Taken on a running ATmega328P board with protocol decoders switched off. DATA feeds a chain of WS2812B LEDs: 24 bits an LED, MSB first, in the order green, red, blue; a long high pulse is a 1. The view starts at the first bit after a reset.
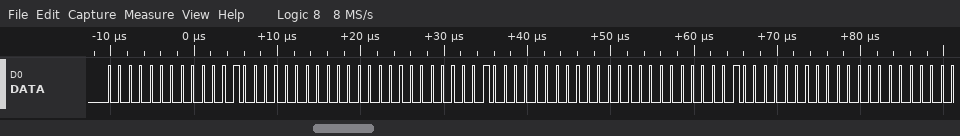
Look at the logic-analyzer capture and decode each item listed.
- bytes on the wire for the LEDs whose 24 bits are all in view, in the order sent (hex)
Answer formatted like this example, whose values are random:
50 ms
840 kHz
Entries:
00 08 00 00 08 00 00 08 00
